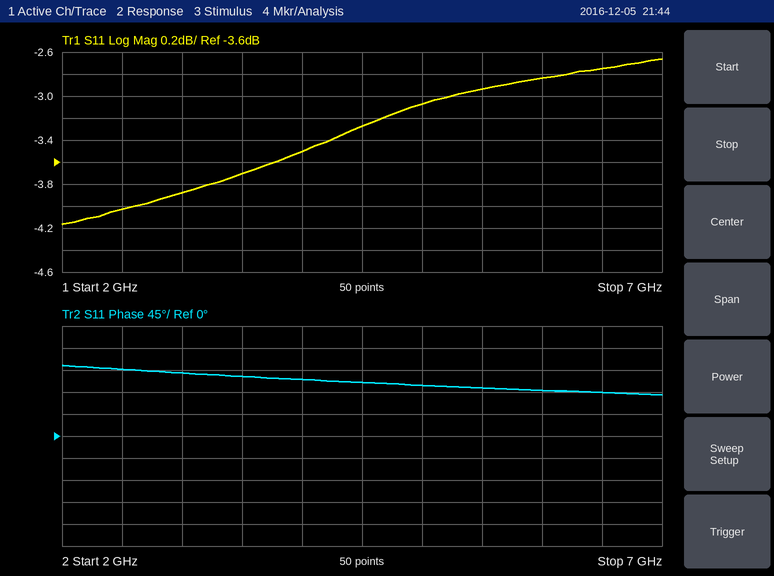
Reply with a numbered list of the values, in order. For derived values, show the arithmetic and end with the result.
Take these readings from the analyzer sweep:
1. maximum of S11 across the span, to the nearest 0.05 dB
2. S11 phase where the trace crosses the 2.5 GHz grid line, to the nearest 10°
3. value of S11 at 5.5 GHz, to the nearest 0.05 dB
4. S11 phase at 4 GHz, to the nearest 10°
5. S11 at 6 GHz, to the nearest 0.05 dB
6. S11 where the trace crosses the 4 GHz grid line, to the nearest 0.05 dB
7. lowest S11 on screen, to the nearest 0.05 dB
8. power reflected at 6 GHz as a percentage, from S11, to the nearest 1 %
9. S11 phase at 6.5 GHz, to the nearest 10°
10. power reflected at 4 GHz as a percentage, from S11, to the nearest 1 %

1. -2.65 dB
2. 140°
3. -2.95 dB
4. 120°
5. -2.85 dB
6. -3.50 dB
7. -4.15 dB
8. 10^(-2.85/10) ≈ 52 %
9. 90°
10. 10^(-3.5/10) ≈ 45 %
